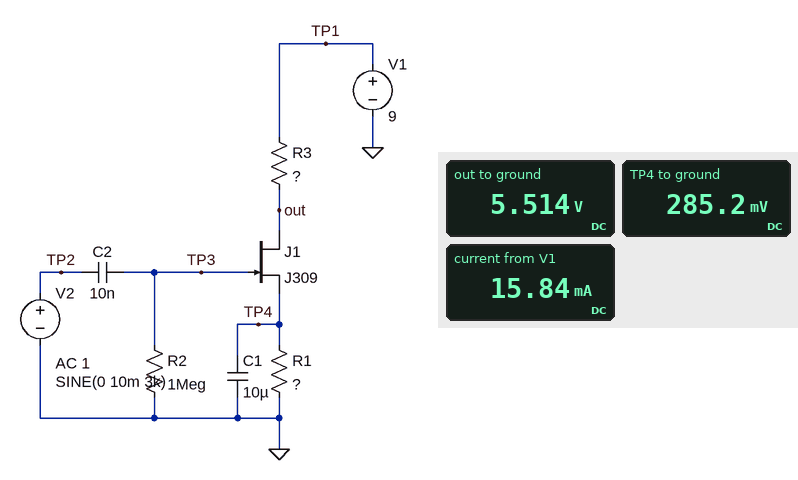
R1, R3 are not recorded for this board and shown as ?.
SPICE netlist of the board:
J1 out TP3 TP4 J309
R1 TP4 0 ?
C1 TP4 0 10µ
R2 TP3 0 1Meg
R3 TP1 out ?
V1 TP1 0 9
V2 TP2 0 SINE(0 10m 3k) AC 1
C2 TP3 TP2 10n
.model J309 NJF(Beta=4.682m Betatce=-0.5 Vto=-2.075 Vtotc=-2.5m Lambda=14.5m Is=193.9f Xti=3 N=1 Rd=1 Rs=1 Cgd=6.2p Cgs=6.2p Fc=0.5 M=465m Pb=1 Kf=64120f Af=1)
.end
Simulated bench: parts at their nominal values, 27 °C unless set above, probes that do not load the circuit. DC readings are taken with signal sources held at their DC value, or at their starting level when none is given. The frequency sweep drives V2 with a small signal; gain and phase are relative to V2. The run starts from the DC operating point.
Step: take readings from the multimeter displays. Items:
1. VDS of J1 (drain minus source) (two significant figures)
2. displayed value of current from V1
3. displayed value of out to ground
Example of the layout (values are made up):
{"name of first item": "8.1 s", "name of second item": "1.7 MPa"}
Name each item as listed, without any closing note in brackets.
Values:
{"VDS of J1 (drain minus source)": "5.2 V", "displayed value of current from V1": "15.84 mA", "displayed value of out to ground": "5.514 V"}
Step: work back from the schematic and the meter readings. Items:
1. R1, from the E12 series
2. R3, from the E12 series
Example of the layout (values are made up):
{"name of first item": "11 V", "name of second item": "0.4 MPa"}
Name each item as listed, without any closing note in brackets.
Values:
{"R1, from the E12 series": "18 Ω", "R3, from the E12 series": "220 Ω"}
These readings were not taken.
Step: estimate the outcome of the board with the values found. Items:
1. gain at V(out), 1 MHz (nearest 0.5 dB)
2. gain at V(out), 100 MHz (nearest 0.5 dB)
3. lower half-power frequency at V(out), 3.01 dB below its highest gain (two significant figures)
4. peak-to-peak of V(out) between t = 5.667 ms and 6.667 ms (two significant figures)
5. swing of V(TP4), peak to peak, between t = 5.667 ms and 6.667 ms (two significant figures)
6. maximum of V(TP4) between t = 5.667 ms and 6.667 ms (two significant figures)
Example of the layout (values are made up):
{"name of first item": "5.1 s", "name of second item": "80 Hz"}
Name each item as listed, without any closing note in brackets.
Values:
{"gain at V(out), 1 MHz": "11.5 dB", "gain at V(out), 100 MHz": "11.0 dB", "lower half-power frequency at V(out), 3.01 dB below its highest gain": "38 Hz", "peak-to-peak of V(out) between t = 5.667 ms and 6.667 ms": "72 mV", "swing of V(TP4), peak to peak, between t = 5.667 ms and 6.667 ms": "1.7 mV", "maximum of V(TP4) between t = 5.667 ms and 6.667 ms": "290 mV"}
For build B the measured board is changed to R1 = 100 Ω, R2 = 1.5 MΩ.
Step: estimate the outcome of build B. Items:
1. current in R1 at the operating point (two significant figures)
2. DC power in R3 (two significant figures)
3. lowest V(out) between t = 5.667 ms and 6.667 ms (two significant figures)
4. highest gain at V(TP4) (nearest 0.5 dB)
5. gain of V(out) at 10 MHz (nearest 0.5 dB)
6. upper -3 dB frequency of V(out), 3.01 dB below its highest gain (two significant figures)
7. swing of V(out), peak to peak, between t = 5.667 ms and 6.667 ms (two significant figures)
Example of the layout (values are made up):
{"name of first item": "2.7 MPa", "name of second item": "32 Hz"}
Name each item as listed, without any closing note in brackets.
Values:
{"current in R1 at the operating point": "8.1 mA", "DC power in R3": "14 mW", "lowest V(out) between t = 5.667 ms and 6.667 ms": "7.2 V", "highest gain at V(TP4)": "-5.5 dB", "gain of V(out) at 10 MHz": "8.5 dB", "upper -3 dB frequency of V(out), 3.01 dB below its highest gain": "400 MHz", "swing of V(out), peak to peak, between t = 5.667 ms and 6.667 ms": "54 mV"}
